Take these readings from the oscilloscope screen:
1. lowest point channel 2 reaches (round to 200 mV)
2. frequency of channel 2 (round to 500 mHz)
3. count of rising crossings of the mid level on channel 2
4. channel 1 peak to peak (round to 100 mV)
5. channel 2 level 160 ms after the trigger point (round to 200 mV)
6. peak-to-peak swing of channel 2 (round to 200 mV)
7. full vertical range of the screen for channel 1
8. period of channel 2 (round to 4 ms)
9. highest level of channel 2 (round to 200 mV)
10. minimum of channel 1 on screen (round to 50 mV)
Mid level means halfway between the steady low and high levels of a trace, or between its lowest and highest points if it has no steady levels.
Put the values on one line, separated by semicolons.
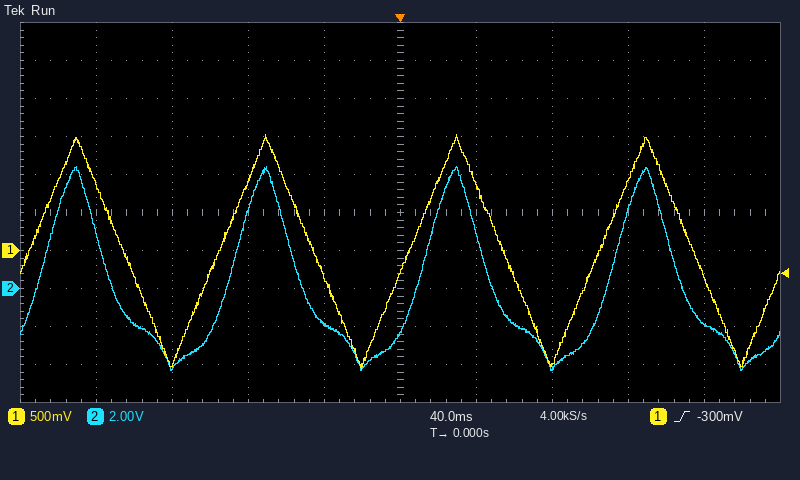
-4.4 V; 10.0 Hz; 4; 3.10 V; -1.8 V; 10.8 V; 5 V; 100 ms; 6.4 V; -1.55 V
